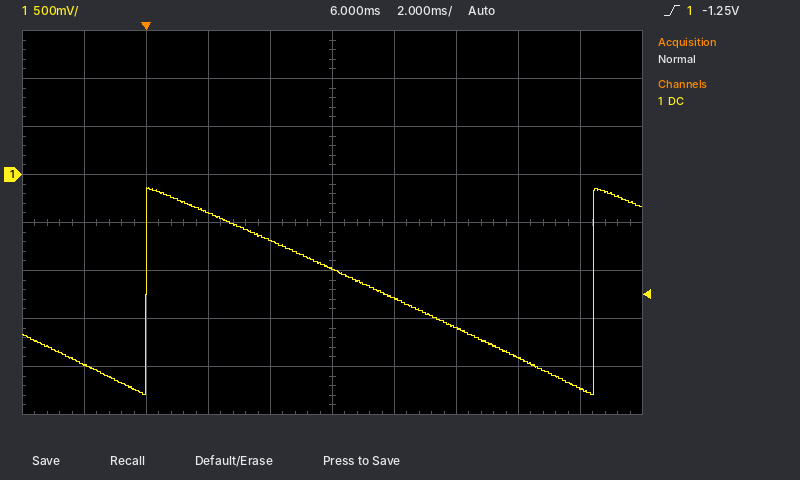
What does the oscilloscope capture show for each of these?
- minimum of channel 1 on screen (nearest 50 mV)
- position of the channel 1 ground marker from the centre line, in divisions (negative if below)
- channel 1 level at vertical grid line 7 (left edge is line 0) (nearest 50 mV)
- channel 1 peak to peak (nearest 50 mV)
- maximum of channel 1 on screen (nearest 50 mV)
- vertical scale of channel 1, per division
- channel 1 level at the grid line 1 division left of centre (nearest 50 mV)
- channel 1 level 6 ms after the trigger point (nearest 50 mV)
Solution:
-2.30 V
+1.0 div
-1.60 V
2.15 V
-150 mV
500 mV
-700 mV
-1.00 V
